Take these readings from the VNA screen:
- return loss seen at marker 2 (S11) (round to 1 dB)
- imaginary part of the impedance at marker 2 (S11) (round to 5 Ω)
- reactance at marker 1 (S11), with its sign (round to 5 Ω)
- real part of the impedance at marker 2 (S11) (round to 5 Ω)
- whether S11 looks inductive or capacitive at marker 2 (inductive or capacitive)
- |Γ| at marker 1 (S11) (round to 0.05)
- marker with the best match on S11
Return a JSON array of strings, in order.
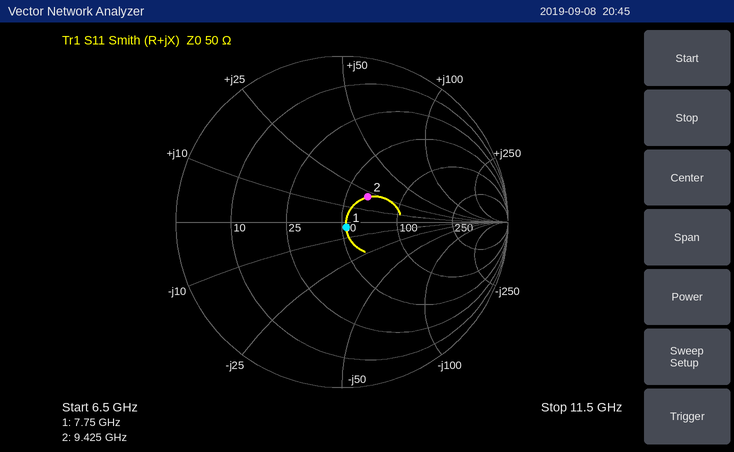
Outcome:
["13 dB", "+20 Ω", "-5 Ω", "65 Ω", "inductive", "0.05", "marker 1"]
